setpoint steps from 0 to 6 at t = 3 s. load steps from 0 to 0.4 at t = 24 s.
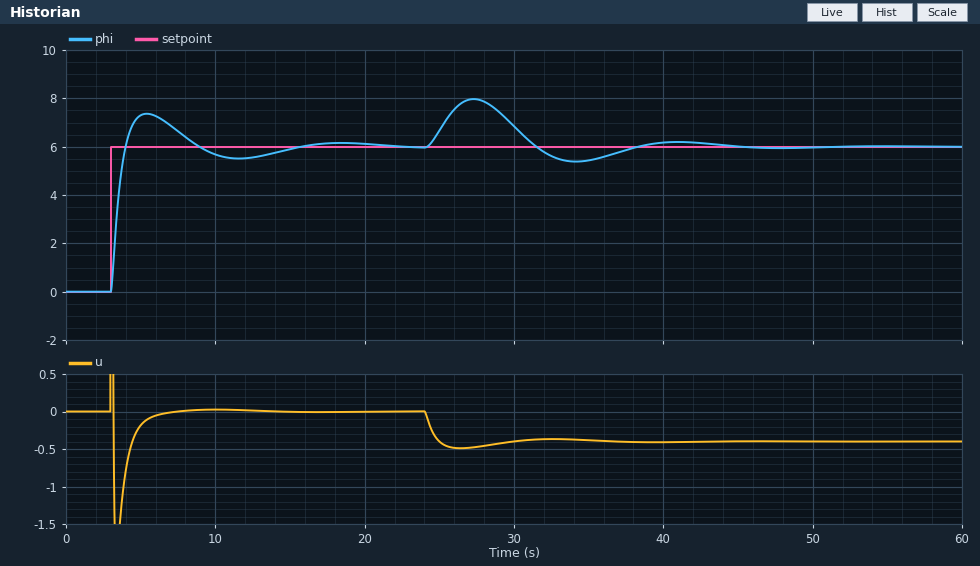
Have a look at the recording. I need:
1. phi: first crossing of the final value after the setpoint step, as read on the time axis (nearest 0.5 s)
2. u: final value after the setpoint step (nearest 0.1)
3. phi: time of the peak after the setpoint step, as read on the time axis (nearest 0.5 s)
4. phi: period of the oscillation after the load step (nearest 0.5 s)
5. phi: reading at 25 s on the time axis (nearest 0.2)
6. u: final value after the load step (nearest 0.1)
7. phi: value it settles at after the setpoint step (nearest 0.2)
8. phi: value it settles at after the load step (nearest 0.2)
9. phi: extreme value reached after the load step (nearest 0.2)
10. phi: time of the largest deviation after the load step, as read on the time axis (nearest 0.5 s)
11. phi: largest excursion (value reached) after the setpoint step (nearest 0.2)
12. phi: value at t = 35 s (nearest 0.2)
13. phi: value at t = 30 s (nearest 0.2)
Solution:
4.0 s
0.0
5.5 s
13.5 s
6.6
-0.4
6.0
6.0
8.0
27.5 s
7.4
5.4
6.8
